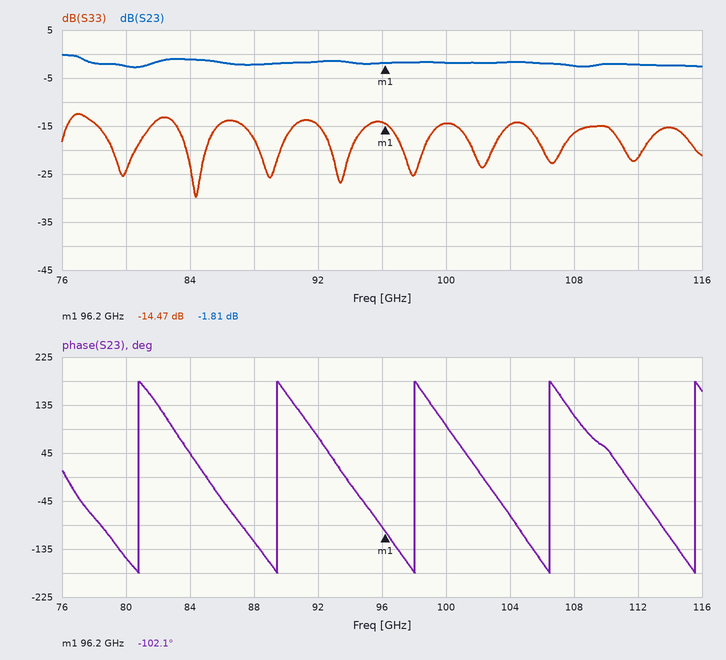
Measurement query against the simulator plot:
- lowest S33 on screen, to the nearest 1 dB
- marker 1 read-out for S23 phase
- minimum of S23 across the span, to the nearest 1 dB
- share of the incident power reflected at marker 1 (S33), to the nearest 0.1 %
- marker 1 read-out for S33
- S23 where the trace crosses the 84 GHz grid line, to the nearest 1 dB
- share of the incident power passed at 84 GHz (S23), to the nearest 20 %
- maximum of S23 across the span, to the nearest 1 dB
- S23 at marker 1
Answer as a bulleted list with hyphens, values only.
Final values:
- -30 dB
- -102.1°
- -3 dB
- 3.6 %
- -14.47 dB
- -1 dB
- 80 %
- 0 dB
- -1.81 dB
